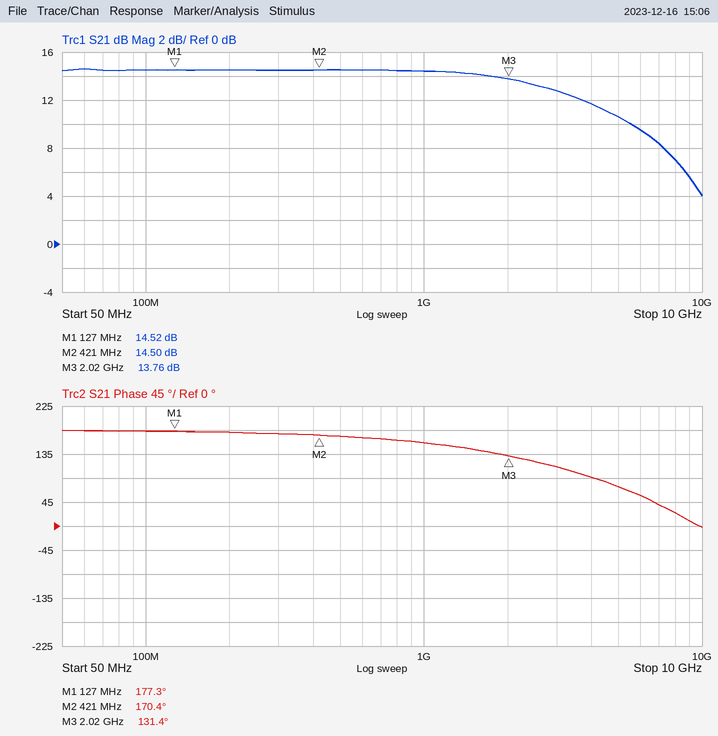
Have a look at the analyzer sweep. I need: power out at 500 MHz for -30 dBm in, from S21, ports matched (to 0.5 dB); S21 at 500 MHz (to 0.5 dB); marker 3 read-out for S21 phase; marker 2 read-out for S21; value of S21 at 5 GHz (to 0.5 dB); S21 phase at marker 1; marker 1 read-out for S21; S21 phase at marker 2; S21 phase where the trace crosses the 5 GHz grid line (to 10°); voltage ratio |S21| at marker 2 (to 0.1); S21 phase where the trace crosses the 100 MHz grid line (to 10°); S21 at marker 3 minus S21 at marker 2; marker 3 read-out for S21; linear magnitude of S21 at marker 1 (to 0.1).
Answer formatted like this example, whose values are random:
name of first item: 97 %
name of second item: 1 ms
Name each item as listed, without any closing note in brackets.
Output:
power out at 500 MHz for -30 dBm in, from S21, ports matched: -15.5 dBm
S21 at 500 MHz: 14.5 dB
marker 3 read-out for S21 phase: 131.4°
marker 2 read-out for S21: 14.50 dB
value of S21 at 5 GHz: 10.5 dB
S21 phase at marker 1: 177.3°
marker 1 read-out for S21: 14.52 dB
S21 phase at marker 2: 170.4°
S21 phase where the trace crosses the 5 GHz grid line: 70°
voltage ratio |S21| at marker 2: 5.3
S21 phase where the trace crosses the 100 MHz grid line: 180°
S21 at marker 3 minus S21 at marker 2: -0.74 dB
marker 3 read-out for S21: 13.76 dB
linear magnitude of S21 at marker 1: 5.3
